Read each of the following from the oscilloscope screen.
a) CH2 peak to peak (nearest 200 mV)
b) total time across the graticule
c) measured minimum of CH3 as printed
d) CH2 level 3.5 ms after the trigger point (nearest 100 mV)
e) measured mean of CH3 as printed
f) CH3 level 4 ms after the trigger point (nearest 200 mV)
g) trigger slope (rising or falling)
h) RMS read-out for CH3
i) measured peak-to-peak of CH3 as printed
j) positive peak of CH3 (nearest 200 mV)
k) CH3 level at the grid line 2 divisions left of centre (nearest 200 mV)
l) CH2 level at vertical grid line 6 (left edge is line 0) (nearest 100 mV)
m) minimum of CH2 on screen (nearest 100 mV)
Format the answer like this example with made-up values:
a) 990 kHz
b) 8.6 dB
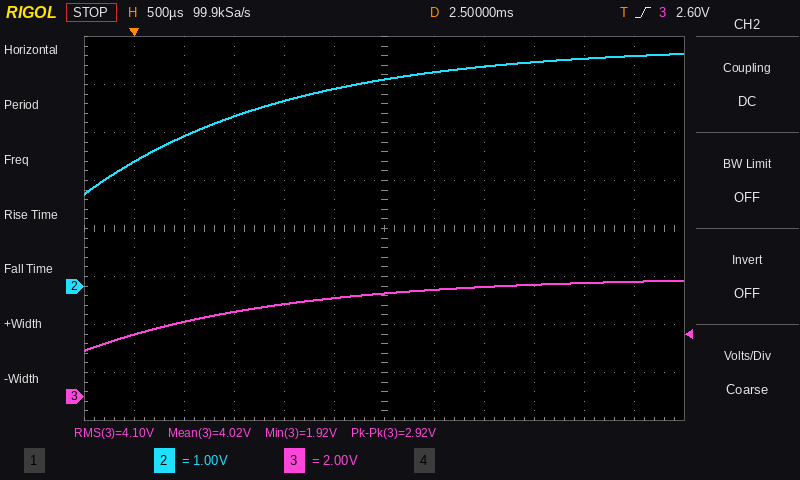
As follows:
a) 3.0 V
b) 6 ms
c) 1.92 V
d) 4.6 V
e) 4.02 V
f) 4.6 V
g) rising
h) 4.10 V
i) 2.92 V
j) 4.8 V
k) 3.8 V
l) 4.3 V
m) 1.9 V
